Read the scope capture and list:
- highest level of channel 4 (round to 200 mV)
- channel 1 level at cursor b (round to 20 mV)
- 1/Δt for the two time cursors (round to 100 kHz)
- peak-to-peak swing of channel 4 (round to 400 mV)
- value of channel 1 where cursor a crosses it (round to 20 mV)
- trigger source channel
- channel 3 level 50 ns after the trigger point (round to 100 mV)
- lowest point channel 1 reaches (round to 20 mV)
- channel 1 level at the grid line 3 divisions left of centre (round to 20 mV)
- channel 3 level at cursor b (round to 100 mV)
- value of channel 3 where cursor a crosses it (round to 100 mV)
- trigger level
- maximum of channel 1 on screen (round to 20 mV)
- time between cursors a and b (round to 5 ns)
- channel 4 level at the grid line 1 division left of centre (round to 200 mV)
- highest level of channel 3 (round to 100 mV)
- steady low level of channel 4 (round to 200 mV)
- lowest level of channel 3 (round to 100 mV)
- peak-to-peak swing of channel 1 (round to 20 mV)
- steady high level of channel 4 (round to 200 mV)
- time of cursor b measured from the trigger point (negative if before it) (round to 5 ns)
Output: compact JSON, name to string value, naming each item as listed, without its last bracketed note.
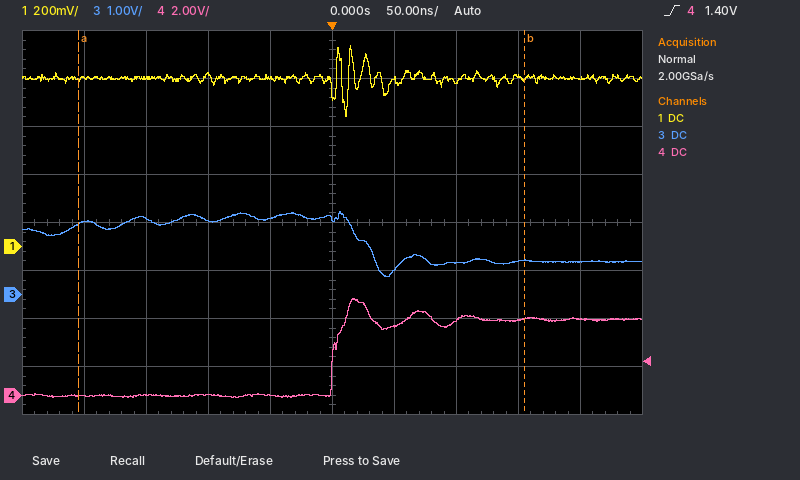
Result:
{"highest level of channel 4": "4.0 V", "channel 1 level at cursor b": "700 mV", "1/Δt for the two time cursors": "2.8 MHz", "peak-to-peak swing of channel 4": "4.0 V", "value of channel 1 where cursor a crosses it": "700 mV", "trigger source channel": "channel 4", "channel 3 level 50 ns after the trigger point": "500 mV", "lowest point channel 1 reaches": "540 mV", "channel 1 level at the grid line 3 divisions left of centre": "700 mV", "channel 3 level at cursor b": "700 mV", "value of channel 3 where cursor a crosses it": "1.5 V", "trigger level": "1.40 V", "maximum of channel 1 on screen": "840 mV", "time between cursors a and b": "360 ns", "channel 4 level at the grid line 1 division left of centre": "0.0 V", "highest level of channel 3": "1.7 V", "steady low level of channel 4": "0.0 V", "lowest level of channel 3": "400 mV", "peak-to-peak swing of channel 1": "300 mV", "steady high level of channel 4": "3.2 V", "time of cursor b measured from the trigger point (negative if before it)": "+155 ns"}
